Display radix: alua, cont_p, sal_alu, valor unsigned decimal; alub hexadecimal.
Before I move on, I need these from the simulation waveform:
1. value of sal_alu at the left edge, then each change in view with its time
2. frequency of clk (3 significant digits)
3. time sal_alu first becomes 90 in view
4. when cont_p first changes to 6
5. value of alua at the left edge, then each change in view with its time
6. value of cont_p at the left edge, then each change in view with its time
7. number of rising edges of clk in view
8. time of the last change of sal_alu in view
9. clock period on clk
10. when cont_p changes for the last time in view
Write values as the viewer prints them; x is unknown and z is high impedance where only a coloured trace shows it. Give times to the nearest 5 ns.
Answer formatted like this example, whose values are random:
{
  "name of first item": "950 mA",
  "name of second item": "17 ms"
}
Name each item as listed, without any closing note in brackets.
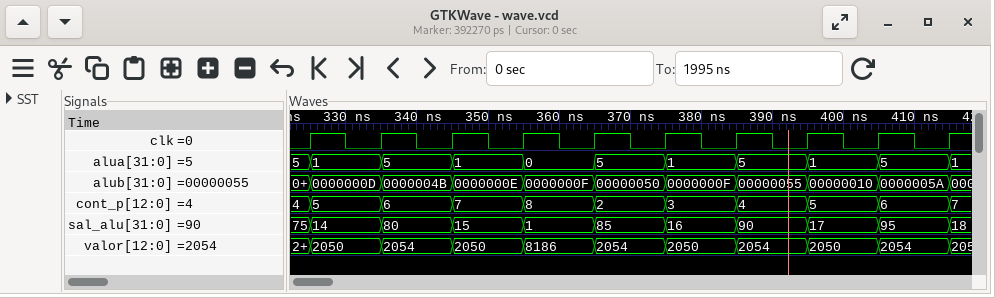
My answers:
{
  "value of sal_alu at the left edge, then each change in view with its time": "75, 14 at 325 ns, 80 at 335 ns, 15 at 345 ns, 1 at 355 ns, 85 at 365 ns, 16 at 375 ns, 90 at 385 ns, 17 at 395 ns, 95 at 405 ns, 18 at 415 ns",
  "frequency of clk": "100 MHz",
  "time sal_alu first becomes 90 in view": "385 ns",
  "when cont_p first changes to 6": "335 ns",
  "value of alua at the left edge, then each change in view with its time": "5, 1 at 325 ns, 5 at 335 ns, 1 at 345 ns, 0 at 355 ns, 5 at 365 ns, 1 at 375 ns, 5 at 385 ns, 1 at 395 ns, 5 at 405 ns, 1 at 415 ns",
  "value of cont_p at the left edge, then each change in view with its time": "4, 5 at 325 ns, 6 at 335 ns, 7 at 345 ns, 8 at 355 ns, 2 at 365 ns, 3 at 375 ns, 4 at 385 ns, 5 at 395 ns, 6 at 405 ns, 7 at 415 ns",
  "number of rising edges of clk in view": "10",
  "time of the last change of sal_alu in view": "415 ns",
  "clock period on clk": "10 ns",
  "when cont_p changes for the last time in view": "415 ns"
}
